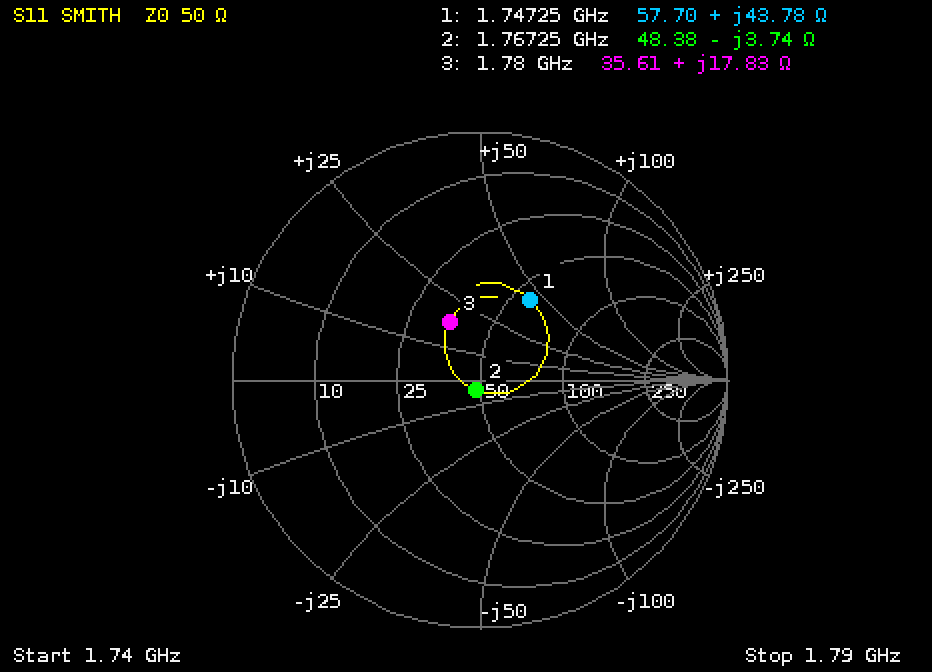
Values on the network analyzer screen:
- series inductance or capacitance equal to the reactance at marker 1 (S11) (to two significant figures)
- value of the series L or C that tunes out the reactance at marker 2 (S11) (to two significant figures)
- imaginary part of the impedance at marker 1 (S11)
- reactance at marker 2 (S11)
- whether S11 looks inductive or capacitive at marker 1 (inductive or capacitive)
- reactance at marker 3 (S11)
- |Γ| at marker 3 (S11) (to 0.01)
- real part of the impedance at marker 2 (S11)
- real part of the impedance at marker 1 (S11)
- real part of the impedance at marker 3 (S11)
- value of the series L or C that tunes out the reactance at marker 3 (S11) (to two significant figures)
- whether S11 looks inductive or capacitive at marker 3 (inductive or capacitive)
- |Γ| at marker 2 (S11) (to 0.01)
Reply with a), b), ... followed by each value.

a) 4.0 nH
b) 340 pH
c) +43.78 Ω
d) -3.74 Ω
e) inductive
f) +17.83 Ω
g) 0.26
h) 48.38 Ω
i) 57.70 Ω
j) 35.61 Ω
k) 5.0 pF
l) inductive
m) 0.04
